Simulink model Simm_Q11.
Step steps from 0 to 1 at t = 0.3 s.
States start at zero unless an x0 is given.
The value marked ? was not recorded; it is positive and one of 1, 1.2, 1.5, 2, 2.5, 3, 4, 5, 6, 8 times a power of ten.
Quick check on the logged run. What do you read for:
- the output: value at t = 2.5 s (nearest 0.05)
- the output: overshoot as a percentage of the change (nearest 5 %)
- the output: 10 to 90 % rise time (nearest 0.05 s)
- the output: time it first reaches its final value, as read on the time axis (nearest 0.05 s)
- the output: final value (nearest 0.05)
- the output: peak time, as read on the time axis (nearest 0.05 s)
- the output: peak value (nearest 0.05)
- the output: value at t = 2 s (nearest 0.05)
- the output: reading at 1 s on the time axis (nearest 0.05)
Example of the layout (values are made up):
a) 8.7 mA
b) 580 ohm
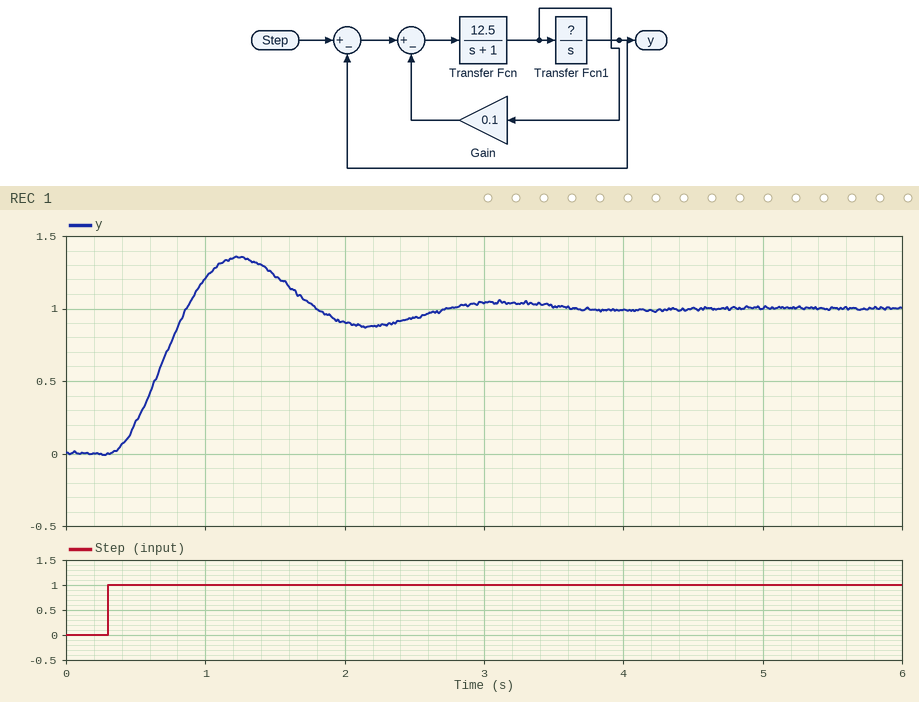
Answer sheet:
a) 0.95
b) 35 %
c) 0.40 s
d) 0.85 s
e) 1.00
f) 1.25 s
g) 1.35
h) 0.90
i) 1.20
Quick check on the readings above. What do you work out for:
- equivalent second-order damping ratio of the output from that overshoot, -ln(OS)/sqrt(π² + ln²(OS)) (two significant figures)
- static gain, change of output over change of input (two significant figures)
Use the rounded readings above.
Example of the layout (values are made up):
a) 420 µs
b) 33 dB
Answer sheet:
a) 0.32
b) 1.0
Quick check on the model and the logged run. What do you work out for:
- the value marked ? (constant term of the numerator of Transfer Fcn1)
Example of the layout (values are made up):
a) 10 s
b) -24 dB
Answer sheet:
a) 1
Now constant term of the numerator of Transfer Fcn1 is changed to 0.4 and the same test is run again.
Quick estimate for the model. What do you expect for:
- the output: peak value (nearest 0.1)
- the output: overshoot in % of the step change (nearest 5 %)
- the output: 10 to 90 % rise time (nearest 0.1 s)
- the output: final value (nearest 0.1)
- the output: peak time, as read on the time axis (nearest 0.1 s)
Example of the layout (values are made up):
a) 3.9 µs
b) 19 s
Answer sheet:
a) 1.2
b) 15 %
c) 0.7 s
d) 1.0
e) 1.9 s
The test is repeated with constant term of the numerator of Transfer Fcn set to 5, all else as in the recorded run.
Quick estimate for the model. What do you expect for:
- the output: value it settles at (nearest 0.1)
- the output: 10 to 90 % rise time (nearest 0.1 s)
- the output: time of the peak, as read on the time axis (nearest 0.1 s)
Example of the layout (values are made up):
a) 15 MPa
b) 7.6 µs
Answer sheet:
a) 1.0
b) 0.6 s
c) 1.8 s
